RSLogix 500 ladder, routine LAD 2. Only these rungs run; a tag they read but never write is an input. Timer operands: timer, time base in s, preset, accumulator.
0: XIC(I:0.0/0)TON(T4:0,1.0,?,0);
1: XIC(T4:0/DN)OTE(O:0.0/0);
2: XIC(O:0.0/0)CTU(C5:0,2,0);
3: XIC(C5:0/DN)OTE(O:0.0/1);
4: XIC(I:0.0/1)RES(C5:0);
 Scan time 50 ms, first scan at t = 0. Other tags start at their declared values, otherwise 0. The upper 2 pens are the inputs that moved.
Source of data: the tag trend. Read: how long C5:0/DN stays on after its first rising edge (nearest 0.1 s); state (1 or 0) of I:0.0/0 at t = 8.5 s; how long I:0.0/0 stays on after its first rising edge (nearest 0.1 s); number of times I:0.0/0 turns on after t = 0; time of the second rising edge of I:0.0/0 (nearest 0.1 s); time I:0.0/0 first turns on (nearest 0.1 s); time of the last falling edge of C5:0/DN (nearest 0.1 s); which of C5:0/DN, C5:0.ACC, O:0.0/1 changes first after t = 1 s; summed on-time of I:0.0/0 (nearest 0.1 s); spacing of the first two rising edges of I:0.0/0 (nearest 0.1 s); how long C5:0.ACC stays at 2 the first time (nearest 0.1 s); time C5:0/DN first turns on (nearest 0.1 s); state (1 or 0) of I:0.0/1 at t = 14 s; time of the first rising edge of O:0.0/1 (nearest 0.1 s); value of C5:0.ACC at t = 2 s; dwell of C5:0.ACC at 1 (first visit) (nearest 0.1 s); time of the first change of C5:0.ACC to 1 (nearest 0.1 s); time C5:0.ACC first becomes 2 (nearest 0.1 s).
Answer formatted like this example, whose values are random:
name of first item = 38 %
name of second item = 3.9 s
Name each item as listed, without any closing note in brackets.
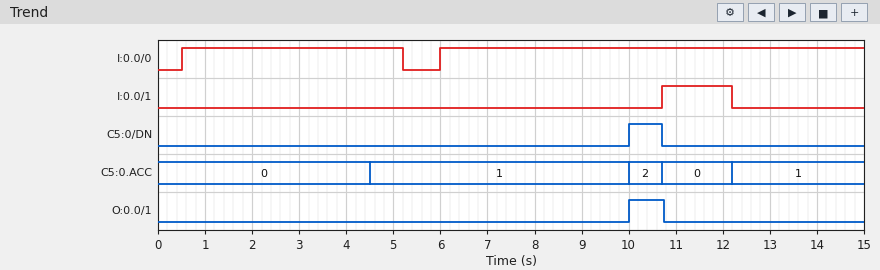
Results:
how long C5:0/DN stays on after its first rising edge = 0.7 s
state (1 or 0) of I:0.0/0 at t = 8.5 s = 1
how long I:0.0/0 stays on after its first rising edge = 4.7 s
number of times I:0.0/0 turns on after t = 0 = 2
time of the second rising edge of I:0.0/0 = 6.0 s
time I:0.0/0 first turns on = 0.5 s
time of the last falling edge of C5:0/DN = 10.7 s
which of C5:0/DN, C5:0.ACC, O:0.0/1 changes first after t = 1 s = C5:0.ACC
summed on-time of I:0.0/0 = 13.7 s
spacing of the first two rising edges of I:0.0/0 = 5.5 s
how long C5:0.ACC stays at 2 the first time = 0.7 s
time C5:0/DN first turns on = 10.0 s
state (1 or 0) of I:0.0/1 at t = 14 s = 0
time of the first rising edge of O:0.0/1 = 10.0 s
value of C5:0.ACC at t = 2 s = 0
dwell of C5:0.ACC at 1 (first visit) = 5.5 s
time of the first change of C5:0.ACC to 1 = 4.5 s
time C5:0.ACC first becomes 2 = 10.0 s
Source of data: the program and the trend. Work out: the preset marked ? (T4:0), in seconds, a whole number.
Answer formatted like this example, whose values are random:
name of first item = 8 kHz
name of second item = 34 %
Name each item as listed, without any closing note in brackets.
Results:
the preset marked ? (T4:0), in seconds, a whole number = 4 s
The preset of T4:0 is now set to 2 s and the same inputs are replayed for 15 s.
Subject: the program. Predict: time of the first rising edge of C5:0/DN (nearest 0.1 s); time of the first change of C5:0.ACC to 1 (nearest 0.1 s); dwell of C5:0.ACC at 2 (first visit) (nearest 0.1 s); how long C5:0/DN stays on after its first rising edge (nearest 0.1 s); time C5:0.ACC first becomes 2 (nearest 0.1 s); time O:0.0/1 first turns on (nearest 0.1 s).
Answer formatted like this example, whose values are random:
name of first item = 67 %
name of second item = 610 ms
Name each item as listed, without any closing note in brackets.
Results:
time of the first rising edge of C5:0/DN = 8.0 s
time of the first change of C5:0.ACC to 1 = 2.5 s
dwell of C5:0.ACC at 2 (first visit) = 2.7 s
how long C5:0/DN stays on after its first rising edge = 2.7 s
time C5:0.ACC first becomes 2 = 8.0 s
time O:0.0/1 first turns on = 8.0 s
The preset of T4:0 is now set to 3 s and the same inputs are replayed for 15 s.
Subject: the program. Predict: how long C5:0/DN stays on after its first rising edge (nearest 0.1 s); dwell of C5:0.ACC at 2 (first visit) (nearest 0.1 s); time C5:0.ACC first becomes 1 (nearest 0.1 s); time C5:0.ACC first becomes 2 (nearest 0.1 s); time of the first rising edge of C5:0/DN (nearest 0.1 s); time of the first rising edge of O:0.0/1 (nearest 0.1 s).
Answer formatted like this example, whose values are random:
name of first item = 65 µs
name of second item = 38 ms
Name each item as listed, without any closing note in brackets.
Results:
how long C5:0/DN stays on after its first rising edge = 1.7 s
dwell of C5:0.ACC at 2 (first visit) = 1.7 s
time C5:0.ACC first becomes 1 = 3.5 s
time C5:0.ACC first becomes 2 = 9.0 s
time of the first rising edge of C5:0/DN = 9.0 s
time of the first rising edge of O:0.0/1 = 9.0 s
